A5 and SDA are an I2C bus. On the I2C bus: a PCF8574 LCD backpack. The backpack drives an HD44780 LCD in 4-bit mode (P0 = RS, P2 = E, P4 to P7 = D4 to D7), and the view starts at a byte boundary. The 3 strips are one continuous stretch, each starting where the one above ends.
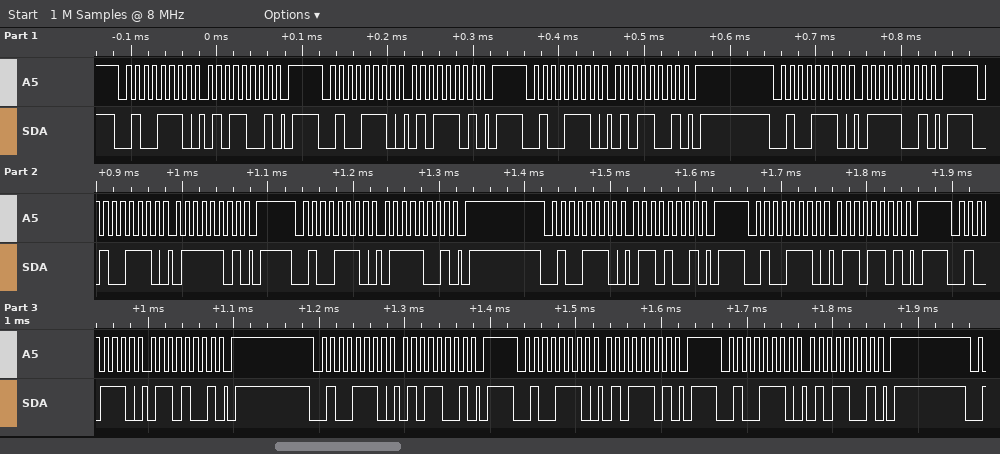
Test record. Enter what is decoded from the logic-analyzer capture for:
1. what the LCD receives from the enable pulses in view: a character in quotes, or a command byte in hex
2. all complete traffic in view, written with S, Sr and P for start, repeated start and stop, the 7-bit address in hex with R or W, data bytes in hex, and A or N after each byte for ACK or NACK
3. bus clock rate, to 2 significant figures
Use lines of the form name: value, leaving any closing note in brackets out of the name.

what the LCD receives from the enable pulses in view: a character in quotes, or a command byte in hex: 'W' 'e'
all complete traffic in view, written with S, Sr and P for start, repeated start and stop, the 7-bit address in hex with R or W, data bytes in hex, and A or N after each byte for ACK or NACK: S 27W A 59 A P S 27W A 5D A P S 27W A 59 A P S 27W A 79 A P S 27W A 7D A P S 27W A 79 A P S 27W A 69 A P S 27W A 6D A P S 27W A 69 A P S 27W A 59 A P S 27W A 5D A P S 27W A 59 A P
bus clock rate, to 2 significant figures: 100 kHz
